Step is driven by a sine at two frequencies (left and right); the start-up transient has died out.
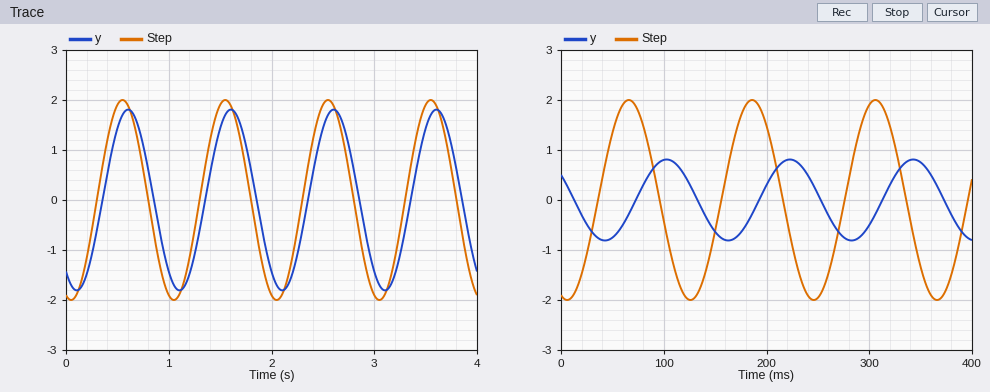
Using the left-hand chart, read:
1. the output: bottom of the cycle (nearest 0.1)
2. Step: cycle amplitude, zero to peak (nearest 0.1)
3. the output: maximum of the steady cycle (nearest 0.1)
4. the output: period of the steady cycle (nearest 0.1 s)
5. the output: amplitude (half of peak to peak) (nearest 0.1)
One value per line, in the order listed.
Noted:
-1.8
2.0
1.8
1.0 s
1.8
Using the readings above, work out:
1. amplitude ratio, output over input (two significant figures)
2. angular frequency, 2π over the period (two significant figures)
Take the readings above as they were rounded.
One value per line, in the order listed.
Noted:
0.90
6.3 rad/s
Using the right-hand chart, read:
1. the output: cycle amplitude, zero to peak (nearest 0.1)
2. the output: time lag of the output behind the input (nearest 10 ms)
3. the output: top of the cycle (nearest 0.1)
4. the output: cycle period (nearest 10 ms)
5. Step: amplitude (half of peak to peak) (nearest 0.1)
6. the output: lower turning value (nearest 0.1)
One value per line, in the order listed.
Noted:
0.8
40 ms
0.8
120 ms
2.0
-0.8
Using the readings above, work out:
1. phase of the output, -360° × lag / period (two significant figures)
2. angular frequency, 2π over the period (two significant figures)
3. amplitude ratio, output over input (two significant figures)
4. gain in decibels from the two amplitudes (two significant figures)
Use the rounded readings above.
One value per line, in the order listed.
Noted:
-120°
0.052 rad/ms
0.40
-8.0 dB
